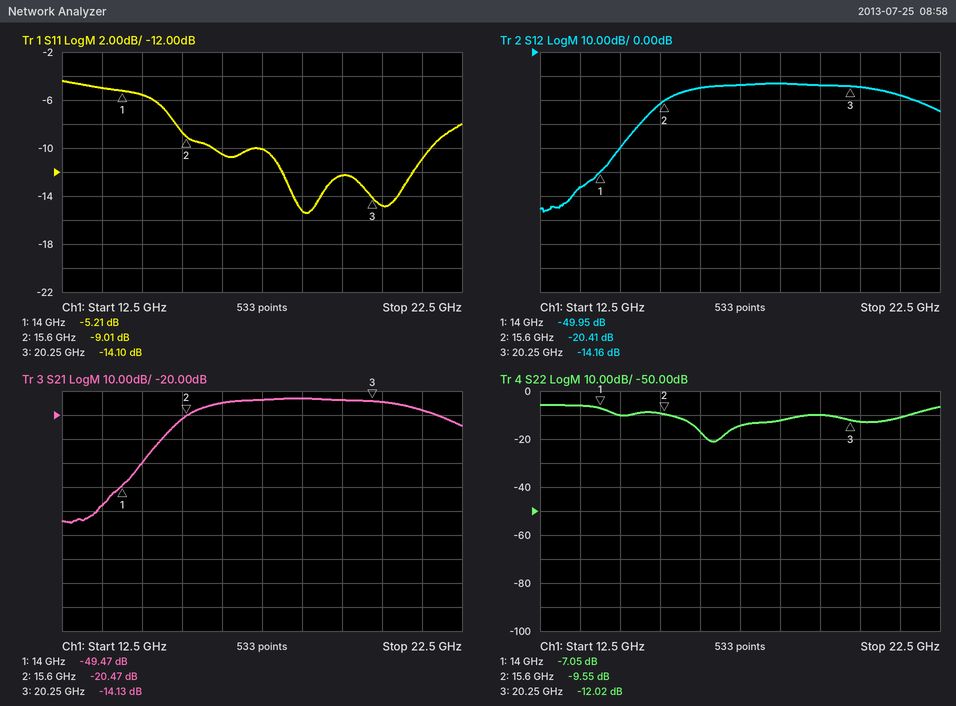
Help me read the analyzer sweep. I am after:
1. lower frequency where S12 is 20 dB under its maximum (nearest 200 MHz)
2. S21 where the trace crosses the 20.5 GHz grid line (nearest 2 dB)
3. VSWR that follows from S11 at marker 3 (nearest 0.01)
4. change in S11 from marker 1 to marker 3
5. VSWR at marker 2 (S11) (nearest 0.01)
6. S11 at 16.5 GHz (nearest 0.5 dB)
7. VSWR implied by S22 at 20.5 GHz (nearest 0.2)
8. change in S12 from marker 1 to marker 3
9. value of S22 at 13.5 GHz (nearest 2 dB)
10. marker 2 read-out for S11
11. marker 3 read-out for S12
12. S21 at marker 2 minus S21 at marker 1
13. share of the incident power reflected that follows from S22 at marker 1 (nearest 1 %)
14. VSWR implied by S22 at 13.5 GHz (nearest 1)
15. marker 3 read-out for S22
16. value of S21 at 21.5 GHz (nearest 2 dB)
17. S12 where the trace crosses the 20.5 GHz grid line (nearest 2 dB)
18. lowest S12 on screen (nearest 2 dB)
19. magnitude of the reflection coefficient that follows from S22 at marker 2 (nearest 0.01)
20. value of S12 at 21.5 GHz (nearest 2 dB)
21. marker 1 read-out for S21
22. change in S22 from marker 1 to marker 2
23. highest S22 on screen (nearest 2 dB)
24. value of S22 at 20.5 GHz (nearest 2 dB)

14.8 GHz
-14 dB
1.49
-8.89 dB
2.10
-10.5 dB
1.6
35.79 dB
-6 dB
-9.01 dB
-14.16 dB
29.00 dB
20 %
3
-12.02 dB
-18 dB
-14 dB
-66 dB
0.33
-18 dB
-49.47 dB
-2.50 dB
-6 dB
-12 dB
